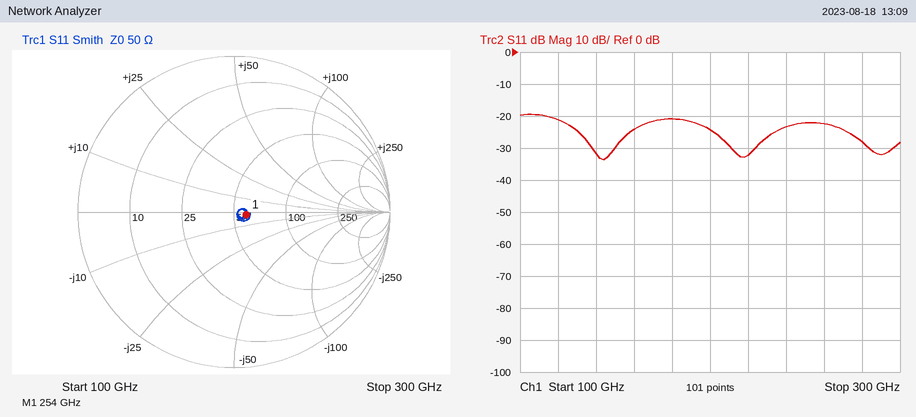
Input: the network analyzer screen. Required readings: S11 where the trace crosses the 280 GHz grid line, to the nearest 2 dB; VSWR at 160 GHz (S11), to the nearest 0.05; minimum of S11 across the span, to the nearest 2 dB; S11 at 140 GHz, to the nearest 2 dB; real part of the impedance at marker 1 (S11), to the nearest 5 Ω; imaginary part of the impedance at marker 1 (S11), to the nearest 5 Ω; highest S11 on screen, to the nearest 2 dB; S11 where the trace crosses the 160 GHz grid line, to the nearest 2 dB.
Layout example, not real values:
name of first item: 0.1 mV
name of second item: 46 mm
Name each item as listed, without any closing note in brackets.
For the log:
S11 where the trace crosses the 280 GHz grid line, to the nearest 2 dB: -28 dB
VSWR at 160 GHz (S11), to the nearest 0.05: 1.15
minimum of S11 across the span, to the nearest 2 dB: -34 dB
S11 at 140 GHz, to the nearest 2 dB: -32 dB
real part of the impedance at marker 1 (S11), to the nearest 5 Ω: 60 Ω
imaginary part of the impedance at marker 1 (S11), to the nearest 5 Ω: 0 Ω
highest S11 on screen, to the nearest 2 dB: -20 dB
S11 where the trace crosses the 160 GHz grid line, to the nearest 2 dB: -24 dB
